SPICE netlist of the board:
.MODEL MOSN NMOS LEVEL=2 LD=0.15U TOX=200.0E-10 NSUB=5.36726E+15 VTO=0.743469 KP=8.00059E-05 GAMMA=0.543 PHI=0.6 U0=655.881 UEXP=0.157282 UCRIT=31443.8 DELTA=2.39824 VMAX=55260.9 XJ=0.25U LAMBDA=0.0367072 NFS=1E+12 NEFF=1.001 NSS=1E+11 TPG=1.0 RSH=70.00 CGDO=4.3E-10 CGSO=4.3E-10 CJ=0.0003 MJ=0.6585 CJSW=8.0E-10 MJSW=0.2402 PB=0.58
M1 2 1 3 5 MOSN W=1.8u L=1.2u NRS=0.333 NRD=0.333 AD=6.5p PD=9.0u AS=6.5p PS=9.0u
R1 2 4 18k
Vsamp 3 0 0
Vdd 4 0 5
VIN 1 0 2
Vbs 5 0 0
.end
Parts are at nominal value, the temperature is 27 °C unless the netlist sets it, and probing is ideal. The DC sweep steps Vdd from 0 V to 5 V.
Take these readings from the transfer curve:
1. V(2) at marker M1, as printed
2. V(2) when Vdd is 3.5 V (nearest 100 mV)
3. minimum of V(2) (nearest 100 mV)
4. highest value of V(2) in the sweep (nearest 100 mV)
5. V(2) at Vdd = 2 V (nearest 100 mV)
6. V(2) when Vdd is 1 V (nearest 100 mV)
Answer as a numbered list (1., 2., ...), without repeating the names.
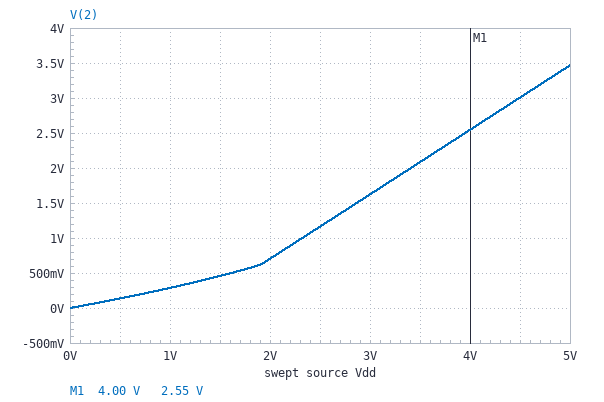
1. 2.55 V
2. 2.1 V
3. 0 V
4. 3.5 V
5. 700 mV
6. 300 mV
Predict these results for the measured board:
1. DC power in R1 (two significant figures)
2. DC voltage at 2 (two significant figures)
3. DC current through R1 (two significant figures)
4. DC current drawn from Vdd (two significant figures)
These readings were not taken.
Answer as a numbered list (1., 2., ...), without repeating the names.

1. 130 µW
2. 3.5 V
3. 85 µA
4. 85 µA
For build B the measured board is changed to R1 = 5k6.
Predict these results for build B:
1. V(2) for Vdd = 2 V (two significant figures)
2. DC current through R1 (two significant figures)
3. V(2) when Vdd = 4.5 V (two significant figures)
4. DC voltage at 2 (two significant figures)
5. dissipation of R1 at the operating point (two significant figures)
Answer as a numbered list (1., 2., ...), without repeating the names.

1. 1.6 V
2. 90 µA
3. 4.0 V
4. 4.5 V
5. 46 µW
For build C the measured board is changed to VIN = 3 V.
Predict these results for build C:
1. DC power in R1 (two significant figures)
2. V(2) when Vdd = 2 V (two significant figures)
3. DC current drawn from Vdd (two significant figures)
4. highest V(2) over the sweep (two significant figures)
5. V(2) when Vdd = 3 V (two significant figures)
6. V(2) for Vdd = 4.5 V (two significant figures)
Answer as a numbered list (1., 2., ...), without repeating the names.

1. 560 µW
2. 390 mV
3. 180 µA
4. 1.8 V
5. 620 mV
6. 1.4 V
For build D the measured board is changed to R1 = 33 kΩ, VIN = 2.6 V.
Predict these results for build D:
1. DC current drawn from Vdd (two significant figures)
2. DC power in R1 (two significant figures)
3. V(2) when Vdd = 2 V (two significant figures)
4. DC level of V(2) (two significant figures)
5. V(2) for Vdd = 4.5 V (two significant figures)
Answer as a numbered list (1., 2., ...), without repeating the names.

1. 130 µA
2. 530 µW
3. 270 mV
4. 800 mV
5. 670 mV
